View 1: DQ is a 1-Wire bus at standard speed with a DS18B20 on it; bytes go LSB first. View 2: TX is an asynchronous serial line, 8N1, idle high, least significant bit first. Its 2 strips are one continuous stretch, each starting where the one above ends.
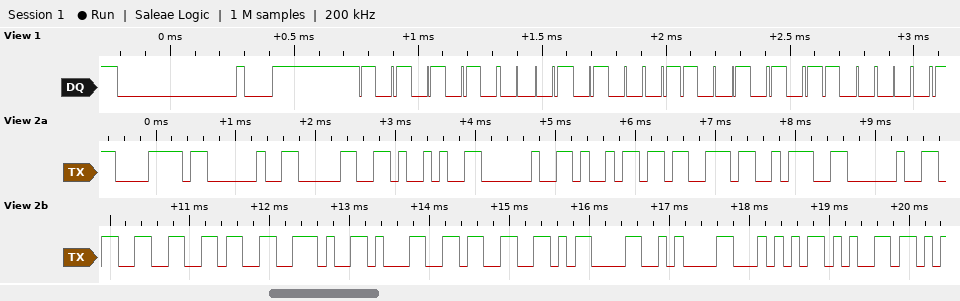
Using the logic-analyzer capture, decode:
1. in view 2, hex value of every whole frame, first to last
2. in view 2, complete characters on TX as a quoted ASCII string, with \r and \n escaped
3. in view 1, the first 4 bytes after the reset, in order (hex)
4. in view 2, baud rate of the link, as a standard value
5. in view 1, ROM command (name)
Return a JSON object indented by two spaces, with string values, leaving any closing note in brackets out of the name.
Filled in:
{
  "in view 2, hex value of every whole frame, first to last": "78 20 30 29 20 69 73 3A 20 33 36 2E 31 33 0D 0A 54 65",
  "in view 2, complete characters on TX as a quoted ASCII string, with \\r and \\n escaped": "\"x 0) is: 36.13\\r\\nTe\"",
  "in view 1, the first 4 bytes after the reset, in order": "55 28 A6 06",
  "in view 2, baud rate of the link, as a standard value": "9600 baud",
  "in view 1, ROM command": "Match ROM"
}
